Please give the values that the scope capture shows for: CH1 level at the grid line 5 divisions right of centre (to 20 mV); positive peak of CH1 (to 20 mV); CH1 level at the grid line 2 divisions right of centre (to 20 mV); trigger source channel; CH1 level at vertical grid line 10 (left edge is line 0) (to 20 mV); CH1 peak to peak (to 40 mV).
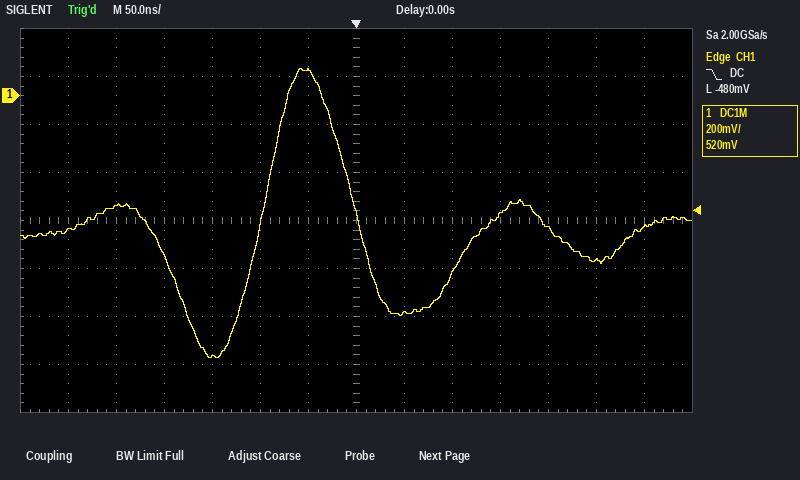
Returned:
-680 mV
120 mV
-740 mV
CH1
-500 mV
1.20 V
